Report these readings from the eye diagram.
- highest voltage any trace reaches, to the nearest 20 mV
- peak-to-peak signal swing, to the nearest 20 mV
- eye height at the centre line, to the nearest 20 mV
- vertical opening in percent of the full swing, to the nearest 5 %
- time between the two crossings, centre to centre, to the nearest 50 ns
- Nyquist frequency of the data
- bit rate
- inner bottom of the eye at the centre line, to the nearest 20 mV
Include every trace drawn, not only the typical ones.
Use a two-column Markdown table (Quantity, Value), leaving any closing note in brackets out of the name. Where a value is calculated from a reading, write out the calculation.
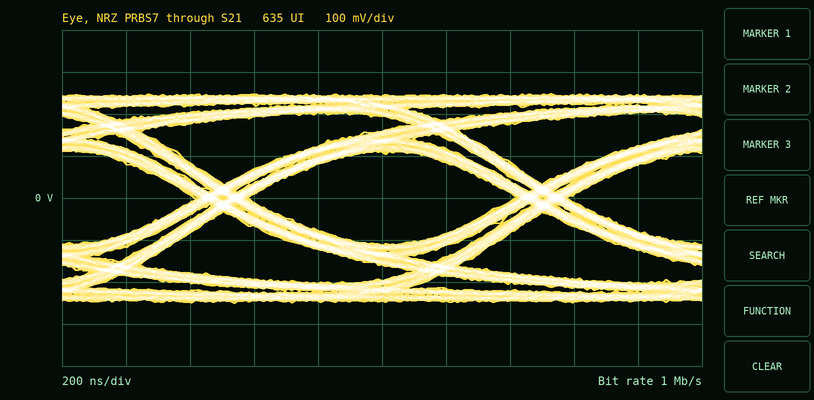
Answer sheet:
| Quantity | Value |
|---|---|
| highest voltage any trace reaches, to the nearest 20 mV | 240 mV |
| peak-to-peak signal swing, to the nearest 20 mV | 500 mV |
| eye height at the centre line, to the nearest 20 mV | 220 mV |
| vertical opening in percent of the full swing, to the nearest 5 % | 220 mV / 500 mV ≈ 44.0 %, so 45 % to the nearest 5 % |
| time between the two crossings, centre to centre, to the nearest 50 ns | 1.00 µs |
| Nyquist frequency of the data | 500 kHz |
| bit rate | 1 Mb/s |
| inner bottom of the eye at the centre line, to the nearest 20 mV | -120 mV |
